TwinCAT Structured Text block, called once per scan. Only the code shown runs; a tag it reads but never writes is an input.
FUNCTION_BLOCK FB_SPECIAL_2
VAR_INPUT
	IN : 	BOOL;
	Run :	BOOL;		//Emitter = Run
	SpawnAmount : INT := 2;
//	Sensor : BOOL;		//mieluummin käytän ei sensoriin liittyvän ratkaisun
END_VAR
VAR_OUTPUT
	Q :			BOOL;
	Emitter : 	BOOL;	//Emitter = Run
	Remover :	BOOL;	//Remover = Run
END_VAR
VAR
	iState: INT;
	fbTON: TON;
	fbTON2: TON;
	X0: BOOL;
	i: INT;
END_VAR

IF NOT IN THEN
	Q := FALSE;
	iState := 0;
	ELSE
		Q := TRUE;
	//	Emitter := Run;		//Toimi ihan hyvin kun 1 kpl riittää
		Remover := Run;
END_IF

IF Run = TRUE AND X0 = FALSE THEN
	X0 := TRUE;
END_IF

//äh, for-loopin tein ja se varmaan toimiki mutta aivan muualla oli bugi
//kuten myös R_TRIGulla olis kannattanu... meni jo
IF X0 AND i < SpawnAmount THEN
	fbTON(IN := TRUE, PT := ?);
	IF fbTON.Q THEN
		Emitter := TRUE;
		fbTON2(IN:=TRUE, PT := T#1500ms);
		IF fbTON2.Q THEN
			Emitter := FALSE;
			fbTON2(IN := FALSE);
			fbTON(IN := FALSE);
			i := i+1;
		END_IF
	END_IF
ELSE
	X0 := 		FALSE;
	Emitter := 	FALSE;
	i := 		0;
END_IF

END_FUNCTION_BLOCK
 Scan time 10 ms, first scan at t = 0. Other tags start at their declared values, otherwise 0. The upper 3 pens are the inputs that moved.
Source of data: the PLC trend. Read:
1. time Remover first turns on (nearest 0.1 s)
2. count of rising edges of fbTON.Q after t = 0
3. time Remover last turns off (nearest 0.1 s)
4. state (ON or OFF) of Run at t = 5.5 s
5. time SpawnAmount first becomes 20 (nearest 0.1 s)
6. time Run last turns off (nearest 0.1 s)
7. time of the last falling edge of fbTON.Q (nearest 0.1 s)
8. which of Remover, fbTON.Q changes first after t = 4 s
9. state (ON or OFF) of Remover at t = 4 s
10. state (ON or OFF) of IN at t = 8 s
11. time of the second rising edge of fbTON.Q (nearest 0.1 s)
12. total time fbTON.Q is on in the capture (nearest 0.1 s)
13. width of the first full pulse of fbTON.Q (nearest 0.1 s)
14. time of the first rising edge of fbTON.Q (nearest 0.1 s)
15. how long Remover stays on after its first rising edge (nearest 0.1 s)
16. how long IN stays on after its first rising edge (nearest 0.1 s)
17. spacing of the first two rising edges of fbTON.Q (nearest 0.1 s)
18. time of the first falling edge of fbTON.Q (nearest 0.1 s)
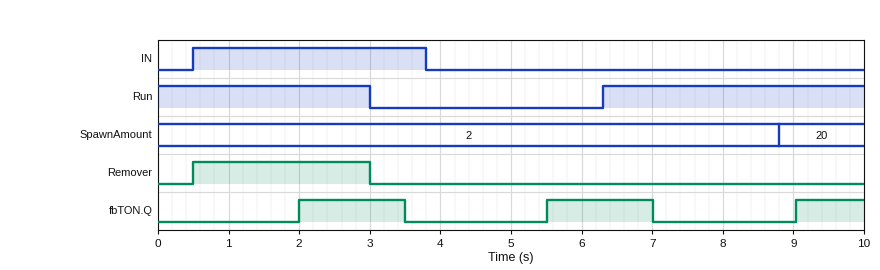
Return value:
0.5 s
3
3.0 s
OFF
8.8 s
3.0 s
7.0 s
fbTON.Q
OFF
OFF
5.5 s
4.0 s
1.5 s
2.0 s
2.5 s
3.3 s
3.5 s
3.5 s
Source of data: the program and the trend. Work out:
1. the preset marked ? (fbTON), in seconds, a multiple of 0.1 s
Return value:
2.0 s
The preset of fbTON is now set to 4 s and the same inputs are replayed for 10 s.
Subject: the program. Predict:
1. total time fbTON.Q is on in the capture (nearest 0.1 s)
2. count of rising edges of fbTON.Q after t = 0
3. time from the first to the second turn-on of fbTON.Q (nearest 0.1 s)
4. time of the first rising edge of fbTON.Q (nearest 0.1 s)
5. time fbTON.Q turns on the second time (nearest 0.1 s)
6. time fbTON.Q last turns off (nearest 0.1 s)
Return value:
2.0 s
2
5.5 s
4.0 s
9.5 s
5.5 s
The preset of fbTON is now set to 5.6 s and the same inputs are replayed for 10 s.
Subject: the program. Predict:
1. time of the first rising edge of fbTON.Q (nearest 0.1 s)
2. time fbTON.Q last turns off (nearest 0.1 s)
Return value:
5.6 s
7.1 s
